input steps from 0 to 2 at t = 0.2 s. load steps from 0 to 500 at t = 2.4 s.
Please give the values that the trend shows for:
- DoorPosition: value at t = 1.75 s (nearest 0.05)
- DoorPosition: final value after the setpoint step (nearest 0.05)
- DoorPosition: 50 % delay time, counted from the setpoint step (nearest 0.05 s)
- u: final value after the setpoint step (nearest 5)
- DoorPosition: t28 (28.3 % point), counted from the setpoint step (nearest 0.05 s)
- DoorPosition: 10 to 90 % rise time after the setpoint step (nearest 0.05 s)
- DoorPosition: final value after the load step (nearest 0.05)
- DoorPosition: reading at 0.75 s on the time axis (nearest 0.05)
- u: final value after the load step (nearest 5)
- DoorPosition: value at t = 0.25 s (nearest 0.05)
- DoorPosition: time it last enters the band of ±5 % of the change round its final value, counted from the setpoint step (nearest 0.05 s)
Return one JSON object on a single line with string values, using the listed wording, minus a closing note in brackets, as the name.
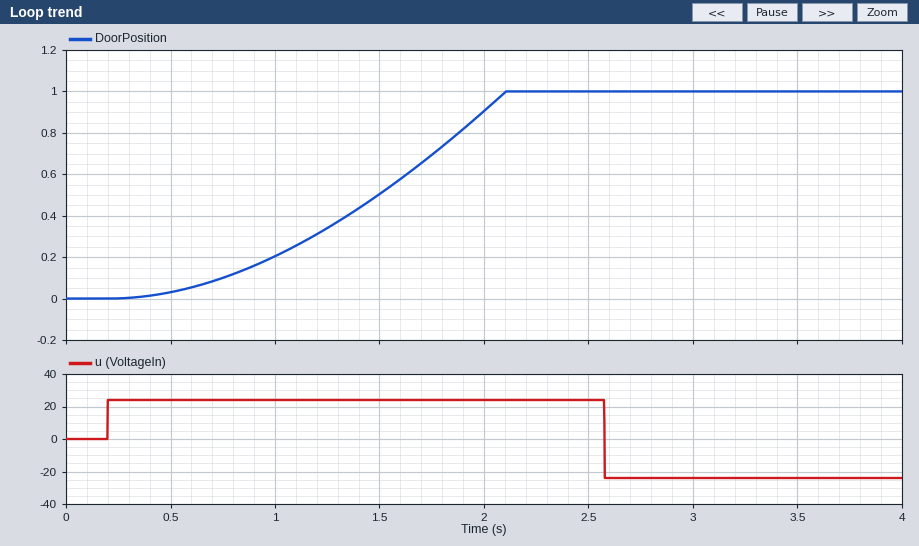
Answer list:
{"DoorPosition: value at t = 1.75 s": "0.70", "DoorPosition: final value after the setpoint step": "1.00", "DoorPosition: 50 % delay time, counted from the setpoint step": "1.30 s", "u: final value after the setpoint step": "25", "DoorPosition: t28 (28.3 % point), counted from the setpoint step": "0.95 s", "DoorPosition: 10 to 90 % rise time after the setpoint step": "1.25 s", "DoorPosition: final value after the load step": "1.00", "DoorPosition: reading at 0.75 s on the time axis": "0.10", "u: final value after the load step": "-25", "DoorPosition: value at t = 0.25 s": "0.00", "DoorPosition: time it last enters the band of ±5 % of the change round its final value, counted from the setpoint step": "1.85 s"}
